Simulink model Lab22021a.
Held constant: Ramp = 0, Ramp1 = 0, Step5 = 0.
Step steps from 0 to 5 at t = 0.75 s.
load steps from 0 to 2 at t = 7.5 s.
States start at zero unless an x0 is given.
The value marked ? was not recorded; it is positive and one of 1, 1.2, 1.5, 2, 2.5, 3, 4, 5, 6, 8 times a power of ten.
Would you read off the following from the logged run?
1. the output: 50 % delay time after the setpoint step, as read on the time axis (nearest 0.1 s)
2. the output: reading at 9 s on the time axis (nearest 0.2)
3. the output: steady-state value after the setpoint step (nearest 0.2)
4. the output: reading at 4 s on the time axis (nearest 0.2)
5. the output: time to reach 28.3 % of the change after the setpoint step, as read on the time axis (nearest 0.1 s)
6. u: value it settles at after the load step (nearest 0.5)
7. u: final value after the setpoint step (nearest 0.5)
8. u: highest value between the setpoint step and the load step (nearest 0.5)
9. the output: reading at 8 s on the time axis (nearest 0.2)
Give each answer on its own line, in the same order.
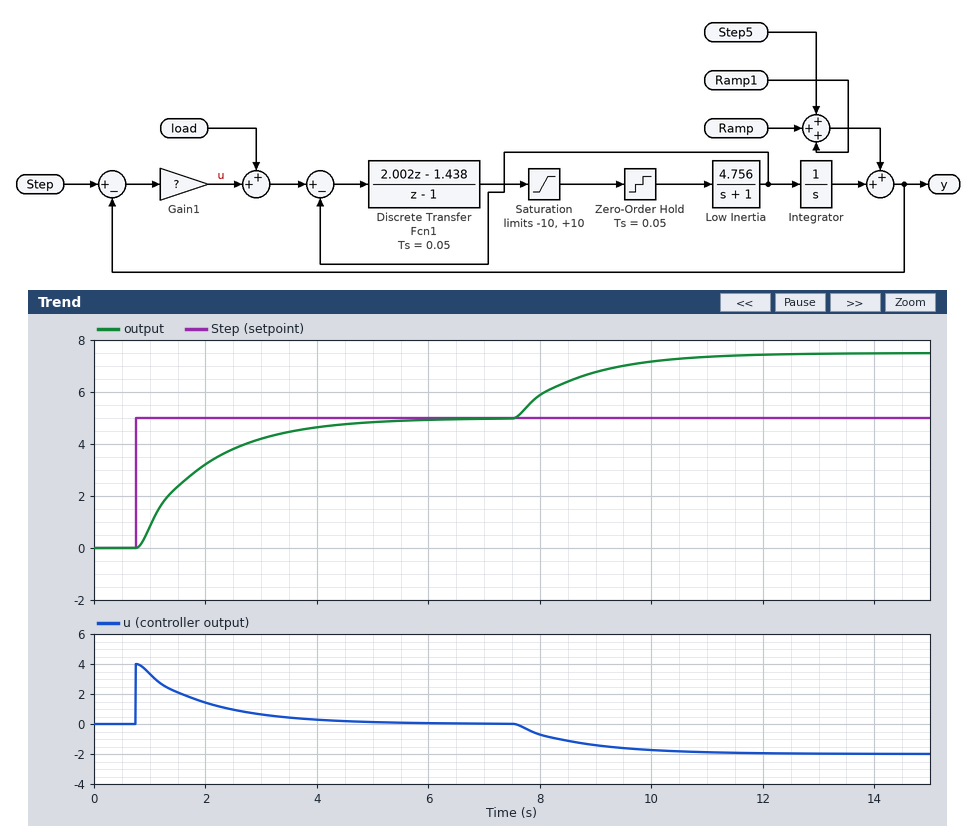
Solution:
1.6 s
6.8
5.0
4.6
1.1 s
-2.0
0.0
4.0
5.8
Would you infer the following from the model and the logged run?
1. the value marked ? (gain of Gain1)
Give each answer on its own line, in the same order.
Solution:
0.8
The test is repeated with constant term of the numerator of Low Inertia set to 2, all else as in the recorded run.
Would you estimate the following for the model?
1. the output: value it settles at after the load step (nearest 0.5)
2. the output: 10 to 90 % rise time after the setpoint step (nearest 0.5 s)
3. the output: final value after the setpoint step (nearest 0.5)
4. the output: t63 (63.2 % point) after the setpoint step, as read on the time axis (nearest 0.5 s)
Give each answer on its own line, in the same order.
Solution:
7.5
2.5 s
5.0
2.0 s
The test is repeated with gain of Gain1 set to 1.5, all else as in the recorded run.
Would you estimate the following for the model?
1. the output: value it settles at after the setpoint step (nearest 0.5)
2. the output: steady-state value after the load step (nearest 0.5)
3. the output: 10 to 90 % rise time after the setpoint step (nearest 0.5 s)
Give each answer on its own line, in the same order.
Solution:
5.0
6.5
1.5 s
